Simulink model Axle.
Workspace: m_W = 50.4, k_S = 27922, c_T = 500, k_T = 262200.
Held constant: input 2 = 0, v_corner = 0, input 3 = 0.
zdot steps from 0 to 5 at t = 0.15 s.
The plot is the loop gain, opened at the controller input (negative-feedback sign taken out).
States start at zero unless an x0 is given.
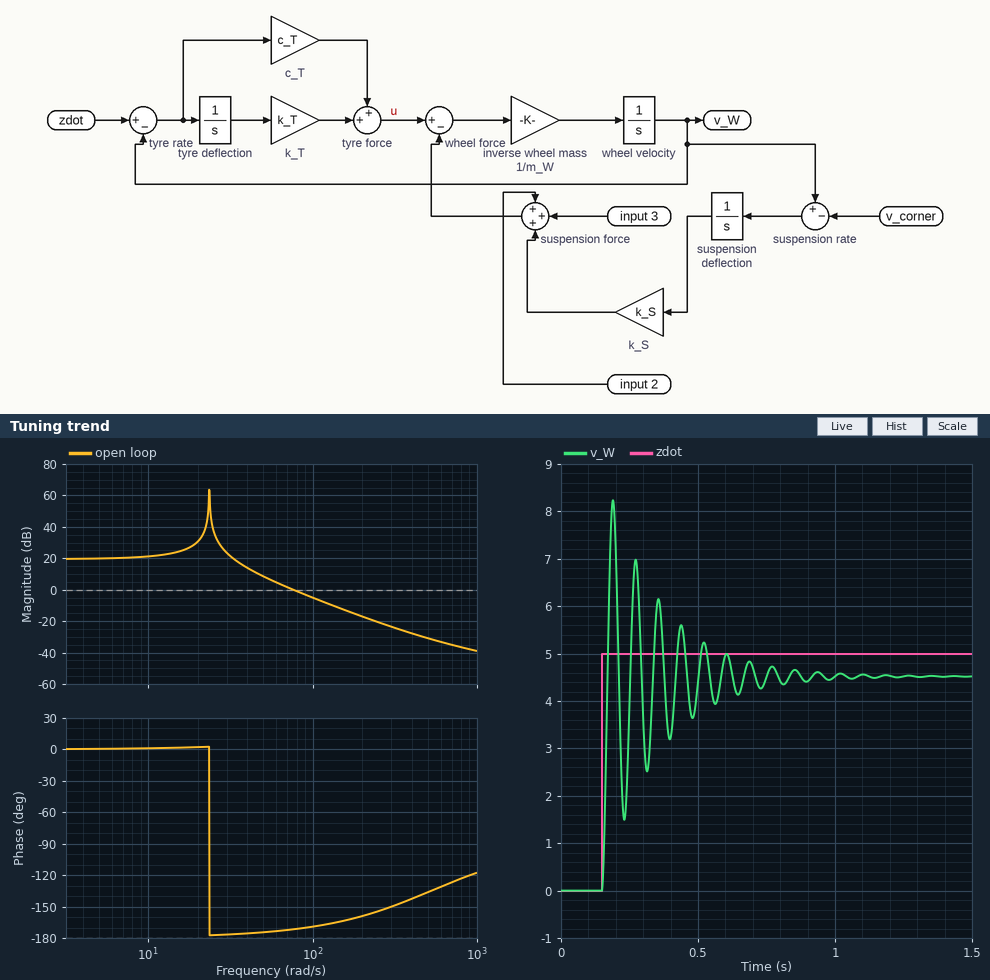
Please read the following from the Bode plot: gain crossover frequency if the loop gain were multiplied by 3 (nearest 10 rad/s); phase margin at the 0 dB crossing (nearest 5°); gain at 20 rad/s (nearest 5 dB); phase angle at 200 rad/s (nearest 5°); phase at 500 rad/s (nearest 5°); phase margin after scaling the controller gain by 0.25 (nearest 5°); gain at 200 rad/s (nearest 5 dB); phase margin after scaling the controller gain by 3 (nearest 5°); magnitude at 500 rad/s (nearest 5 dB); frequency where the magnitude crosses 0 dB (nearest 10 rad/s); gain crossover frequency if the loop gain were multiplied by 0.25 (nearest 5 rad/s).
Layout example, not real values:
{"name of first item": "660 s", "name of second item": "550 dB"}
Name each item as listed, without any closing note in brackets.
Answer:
{"gain crossover frequency if the loop gain were multiplied by 3": "130 rad/s", "phase margin at the 0 dB crossing": "10°", "gain at 20 rad/s": "30 dB", "phase angle at 200 rad/s": "-160°", "phase at 500 rad/s": "-135°", "phase margin after scaling the controller gain by 0.25": "5°", "gain at 200 rad/s": "-15 dB", "phase margin after scaling the controller gain by 3": "15°", "magnitude at 500 rad/s": "-30 dB", "frequency where the magnitude crosses 0 dB": "80 rad/s", "gain crossover frequency if the loop gain were multiplied by 0.25": "45 rad/s"}
